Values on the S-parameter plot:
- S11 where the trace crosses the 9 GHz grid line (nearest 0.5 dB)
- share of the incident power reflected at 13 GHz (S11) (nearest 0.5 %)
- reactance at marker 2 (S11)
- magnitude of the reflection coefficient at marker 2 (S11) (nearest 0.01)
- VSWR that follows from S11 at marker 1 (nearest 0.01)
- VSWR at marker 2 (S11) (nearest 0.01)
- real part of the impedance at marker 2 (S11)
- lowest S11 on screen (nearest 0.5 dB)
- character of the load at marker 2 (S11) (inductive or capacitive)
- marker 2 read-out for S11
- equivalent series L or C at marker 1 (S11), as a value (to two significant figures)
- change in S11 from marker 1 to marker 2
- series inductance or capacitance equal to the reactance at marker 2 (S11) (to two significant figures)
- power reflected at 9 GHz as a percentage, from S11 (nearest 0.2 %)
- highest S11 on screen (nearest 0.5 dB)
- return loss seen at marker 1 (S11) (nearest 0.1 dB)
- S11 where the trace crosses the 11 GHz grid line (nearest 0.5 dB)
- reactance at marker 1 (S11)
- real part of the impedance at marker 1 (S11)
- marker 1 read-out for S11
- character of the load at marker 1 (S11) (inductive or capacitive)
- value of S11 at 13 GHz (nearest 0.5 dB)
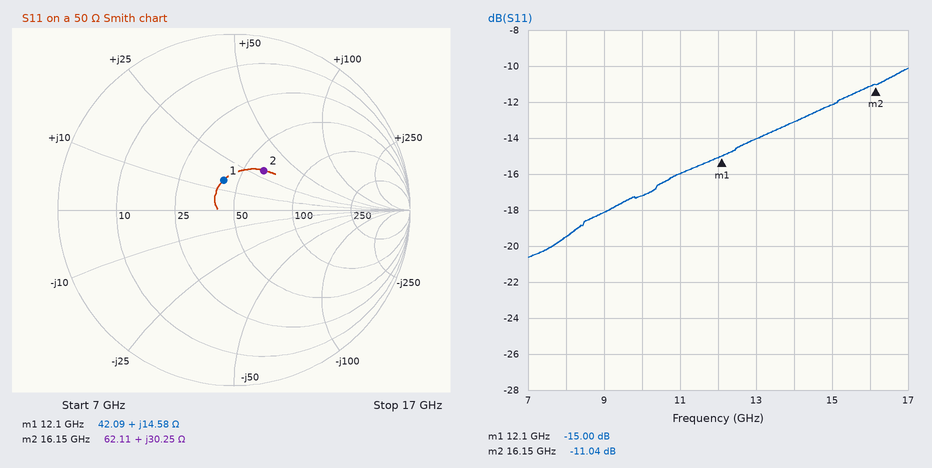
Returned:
-18.0 dB
4.0 %
+30.25 Ω
0.28
1.43
1.78
62.11 Ω
-20.5 dB
inductive
-11.04 dB
190 pH
3.96 dB
300 pH
1.6 %
-10.0 dB
15.0 dB
-16.0 dB
+14.58 Ω
42.09 Ω
-15.00 dB
inductive
-14.0 dB
